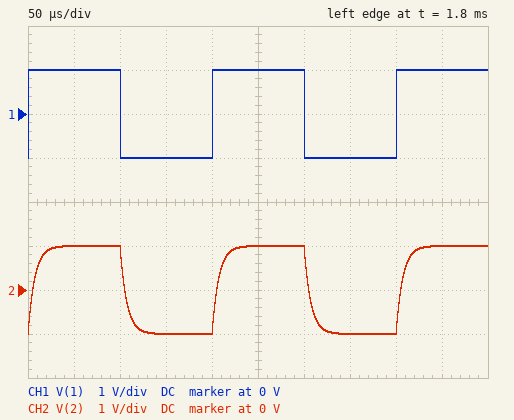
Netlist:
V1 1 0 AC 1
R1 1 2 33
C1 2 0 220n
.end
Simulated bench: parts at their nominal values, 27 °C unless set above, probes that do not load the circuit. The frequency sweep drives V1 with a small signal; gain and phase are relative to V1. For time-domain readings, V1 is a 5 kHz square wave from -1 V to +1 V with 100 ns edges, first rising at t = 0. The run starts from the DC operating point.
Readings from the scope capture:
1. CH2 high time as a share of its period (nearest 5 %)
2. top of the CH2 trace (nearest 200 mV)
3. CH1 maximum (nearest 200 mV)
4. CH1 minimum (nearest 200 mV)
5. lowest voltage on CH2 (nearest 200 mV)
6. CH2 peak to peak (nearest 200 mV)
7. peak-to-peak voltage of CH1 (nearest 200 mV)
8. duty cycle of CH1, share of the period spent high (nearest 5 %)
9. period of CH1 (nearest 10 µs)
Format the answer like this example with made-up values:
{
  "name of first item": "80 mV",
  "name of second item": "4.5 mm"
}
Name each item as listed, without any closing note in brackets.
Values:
{
  "CH2 high time as a share of its period": "50 %",
  "top of the CH2 trace": "1.0 V",
  "CH1 maximum": "1.0 V",
  "CH1 minimum": "-1.0 V",
  "lowest voltage on CH2": "-1.0 V",
  "CH2 peak to peak": "2.0 V",
  "peak-to-peak voltage of CH1": "2.0 V",
  "duty cycle of CH1, share of the period spent high": "50 %",
  "period of CH1": "200 µs"
}
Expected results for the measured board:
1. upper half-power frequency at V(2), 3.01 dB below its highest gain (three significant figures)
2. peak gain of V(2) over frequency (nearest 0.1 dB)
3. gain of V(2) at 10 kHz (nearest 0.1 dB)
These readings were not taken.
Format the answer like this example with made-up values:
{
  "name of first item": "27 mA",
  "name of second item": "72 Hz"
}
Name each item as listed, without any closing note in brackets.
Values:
{
  "upper half-power frequency at V(2), 3.01 dB below its highest gain": "21.9 kHz",
  "peak gain of V(2) over frequency": "0 dB",
  "gain of V(2) at 10 kHz": "-0.8 dB"
}
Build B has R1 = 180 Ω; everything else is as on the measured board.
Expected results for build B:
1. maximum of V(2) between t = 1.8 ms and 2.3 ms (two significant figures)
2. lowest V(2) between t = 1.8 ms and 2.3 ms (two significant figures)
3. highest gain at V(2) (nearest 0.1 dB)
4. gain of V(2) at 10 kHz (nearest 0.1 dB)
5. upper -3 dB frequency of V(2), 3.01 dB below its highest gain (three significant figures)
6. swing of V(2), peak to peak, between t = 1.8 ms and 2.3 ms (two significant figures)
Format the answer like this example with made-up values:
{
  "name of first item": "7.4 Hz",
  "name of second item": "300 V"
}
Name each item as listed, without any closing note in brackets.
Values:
{
  "maximum of V(2) between t = 1.8 ms and 2.3 ms": "850 mV",
  "lowest V(2) between t = 1.8 ms and 2.3 ms": "-850 mV",
  "highest gain at V(2)": "0 dB",
  "gain of V(2) at 10 kHz": "-8.6 dB",
  "upper -3 dB frequency of V(2), 3.01 dB below its highest gain": "4.02 kHz",
  "swing of V(2), peak to peak, between t = 1.8 ms and 2.3 ms": "1.7 V"
}
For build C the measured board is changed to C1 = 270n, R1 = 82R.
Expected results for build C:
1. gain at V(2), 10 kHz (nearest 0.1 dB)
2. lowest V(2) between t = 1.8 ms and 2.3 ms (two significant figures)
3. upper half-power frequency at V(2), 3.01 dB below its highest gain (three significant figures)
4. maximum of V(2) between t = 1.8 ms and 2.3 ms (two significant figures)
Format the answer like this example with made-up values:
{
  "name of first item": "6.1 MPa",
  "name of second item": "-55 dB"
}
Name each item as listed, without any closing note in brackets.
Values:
{
  "gain at V(2), 10 kHz": "-4.7 dB",
  "lowest V(2) between t = 1.8 ms and 2.3 ms": "-980 mV",
  "upper half-power frequency at V(2), 3.01 dB below its highest gain": "7.19 kHz",
  "maximum of V(2) between t = 1.8 ms and 2.3 ms": "980 mV"
}
